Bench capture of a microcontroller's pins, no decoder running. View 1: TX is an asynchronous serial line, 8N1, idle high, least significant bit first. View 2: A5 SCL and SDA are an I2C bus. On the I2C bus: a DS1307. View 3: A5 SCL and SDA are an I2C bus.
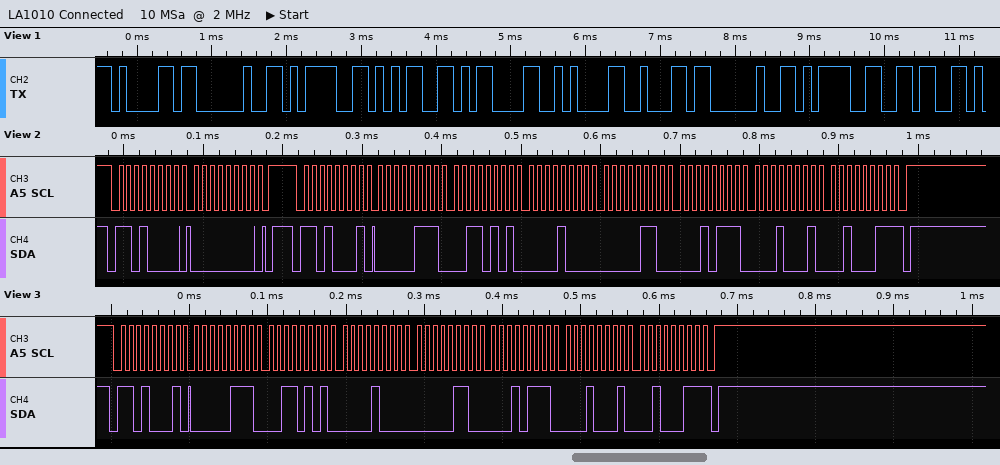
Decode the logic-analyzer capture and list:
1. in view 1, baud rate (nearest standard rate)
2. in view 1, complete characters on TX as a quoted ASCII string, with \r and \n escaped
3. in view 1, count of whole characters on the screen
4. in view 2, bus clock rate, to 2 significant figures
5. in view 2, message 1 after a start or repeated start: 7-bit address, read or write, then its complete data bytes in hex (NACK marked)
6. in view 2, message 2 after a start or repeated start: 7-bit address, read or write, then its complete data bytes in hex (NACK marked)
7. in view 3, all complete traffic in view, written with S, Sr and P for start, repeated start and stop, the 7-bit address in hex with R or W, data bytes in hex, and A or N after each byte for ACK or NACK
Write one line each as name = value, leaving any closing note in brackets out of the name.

in view 1, baud rate = 9600 baud
in view 1, complete characters on TX as a quoted ASCII string, with \r and \n escaped = "a =5\r\nb =6"
in view 1, count of whole characters on the screen = 10
in view 2, bus clock rate, to 2 significant figures = 100 kHz
in view 2, message 1 after a start or repeated start: 7-bit address, read or write, then its complete data bytes in hex = 0x68 write: 00
in view 2, message 2 after a start or repeated start: 7-bit address, read or write, then its complete data bytes in hex = 0x68 read: 07 35 08 06 17 11 23 NACK
in view 3, all complete traffic in view, written with S, Sr and P for start, repeated start and stop, the 7-bit address in hex with R or W, data bytes in hex, and A or N after each byte for ACK or NACK = S 68R A 07 A 35 A 08 A 06 A 17 A 11 A 23 N P
